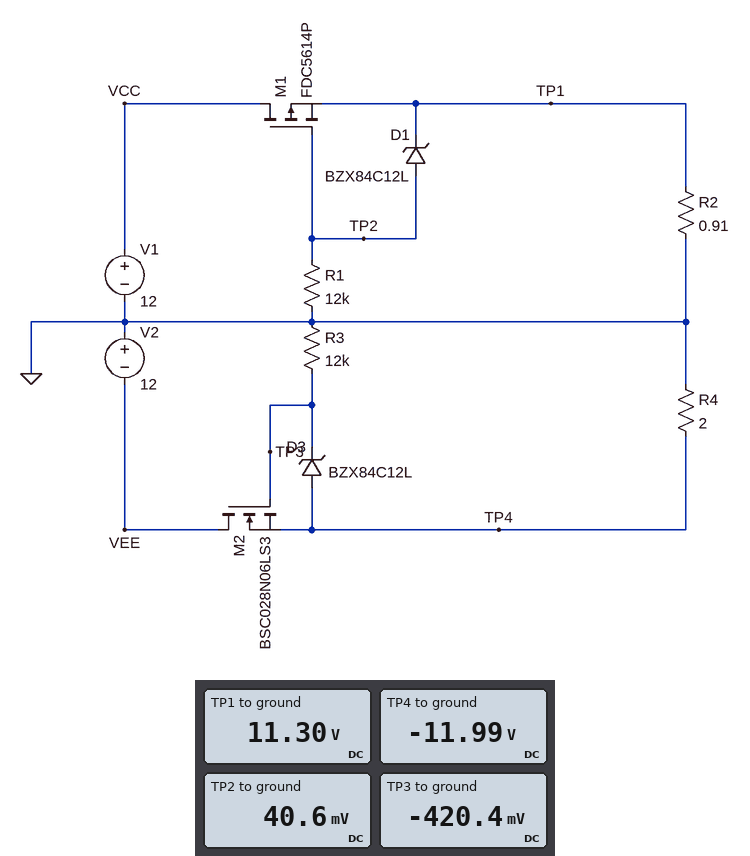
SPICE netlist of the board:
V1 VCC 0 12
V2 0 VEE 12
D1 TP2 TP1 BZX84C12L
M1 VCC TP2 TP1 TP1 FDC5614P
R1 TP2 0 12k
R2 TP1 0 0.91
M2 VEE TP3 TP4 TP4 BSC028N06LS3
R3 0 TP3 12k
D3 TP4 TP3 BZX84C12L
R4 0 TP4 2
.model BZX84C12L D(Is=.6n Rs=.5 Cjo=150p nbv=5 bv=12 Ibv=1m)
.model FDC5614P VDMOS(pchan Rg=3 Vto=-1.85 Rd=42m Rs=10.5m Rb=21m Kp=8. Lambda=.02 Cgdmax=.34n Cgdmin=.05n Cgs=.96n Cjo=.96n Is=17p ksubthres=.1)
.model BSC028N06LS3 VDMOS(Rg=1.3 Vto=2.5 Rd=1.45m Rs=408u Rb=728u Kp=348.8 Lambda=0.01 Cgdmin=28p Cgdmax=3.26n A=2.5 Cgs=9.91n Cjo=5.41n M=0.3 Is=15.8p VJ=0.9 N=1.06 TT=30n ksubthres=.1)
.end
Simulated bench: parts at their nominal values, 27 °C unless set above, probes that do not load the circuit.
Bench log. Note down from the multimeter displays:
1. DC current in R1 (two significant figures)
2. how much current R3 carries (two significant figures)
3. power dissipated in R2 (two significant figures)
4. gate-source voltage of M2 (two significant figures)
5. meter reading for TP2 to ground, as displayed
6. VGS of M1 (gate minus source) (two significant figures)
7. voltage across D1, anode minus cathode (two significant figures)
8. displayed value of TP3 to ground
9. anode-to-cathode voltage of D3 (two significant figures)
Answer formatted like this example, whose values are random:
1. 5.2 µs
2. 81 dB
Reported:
1. 3.4 µA
2. 35 µA
3. 140 W
4. 12 V
5. 40.6 mV
6. -11 V
7. -11 V
8. -420.4 mV
9. -12 V
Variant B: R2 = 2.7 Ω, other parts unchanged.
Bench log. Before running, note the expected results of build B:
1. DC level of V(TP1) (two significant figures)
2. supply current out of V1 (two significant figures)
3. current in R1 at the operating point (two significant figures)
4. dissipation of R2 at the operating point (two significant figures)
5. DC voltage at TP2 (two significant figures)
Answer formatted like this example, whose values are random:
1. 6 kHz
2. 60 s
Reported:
1. 12 V
2. 4.3 A
3. 19 µA
4. 51 W
5. 230 mV
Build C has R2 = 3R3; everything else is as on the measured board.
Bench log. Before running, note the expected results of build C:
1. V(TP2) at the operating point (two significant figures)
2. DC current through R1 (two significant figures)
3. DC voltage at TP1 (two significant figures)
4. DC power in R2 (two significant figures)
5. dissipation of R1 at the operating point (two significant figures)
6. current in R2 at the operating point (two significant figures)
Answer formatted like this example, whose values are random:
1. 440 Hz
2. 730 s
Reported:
1. 260 mV
2. 22 µA
3. 12 V
4. 42 W
5. 5.7 µW
6. 3.6 A
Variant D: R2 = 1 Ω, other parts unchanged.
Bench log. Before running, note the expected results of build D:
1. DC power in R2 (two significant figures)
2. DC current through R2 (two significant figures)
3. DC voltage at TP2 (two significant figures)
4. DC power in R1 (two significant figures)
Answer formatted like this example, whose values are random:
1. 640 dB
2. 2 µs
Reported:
1. 130 W
2. 11 A
3. 47 mV
4. 190 nW
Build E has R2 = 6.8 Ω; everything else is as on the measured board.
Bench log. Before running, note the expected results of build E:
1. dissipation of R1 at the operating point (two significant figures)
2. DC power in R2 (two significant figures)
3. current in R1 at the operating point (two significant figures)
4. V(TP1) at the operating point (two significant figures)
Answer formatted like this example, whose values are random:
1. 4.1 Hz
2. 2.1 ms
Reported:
1. 9.9 µW
2. 21 W
3. 29 µA
4. 12 V
